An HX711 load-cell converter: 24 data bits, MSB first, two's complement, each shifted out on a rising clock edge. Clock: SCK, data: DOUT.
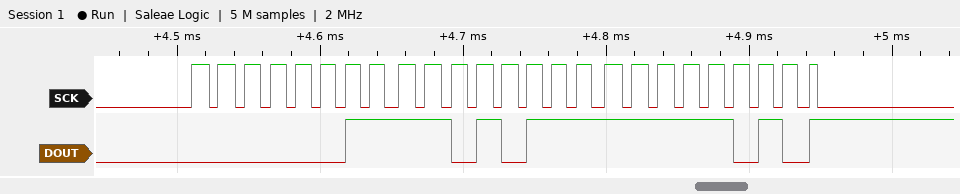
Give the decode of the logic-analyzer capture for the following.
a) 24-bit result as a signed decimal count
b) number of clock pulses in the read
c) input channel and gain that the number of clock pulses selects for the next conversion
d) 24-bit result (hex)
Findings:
251898
25
channel A, gain 128
0x03D7FA
